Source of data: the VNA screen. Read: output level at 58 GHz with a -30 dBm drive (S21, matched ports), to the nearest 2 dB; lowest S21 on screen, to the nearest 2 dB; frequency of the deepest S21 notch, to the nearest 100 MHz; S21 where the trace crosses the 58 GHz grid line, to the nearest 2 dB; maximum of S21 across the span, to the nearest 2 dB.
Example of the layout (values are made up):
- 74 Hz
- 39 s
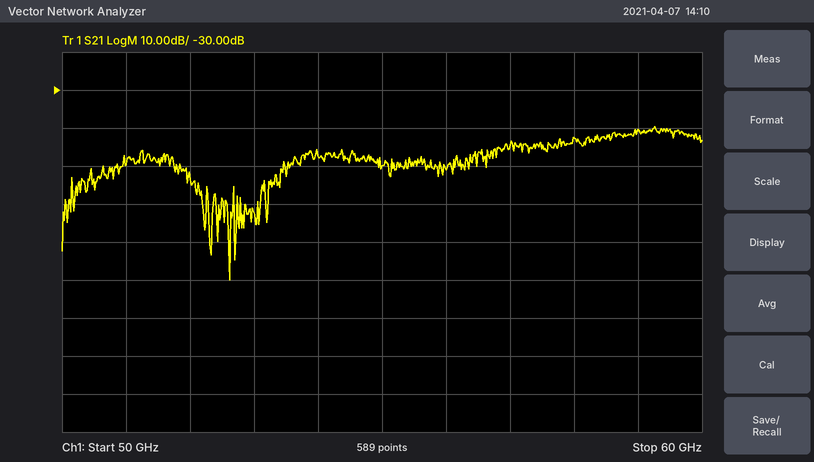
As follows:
- -72 dBm
- -80 dB
- 52.6 GHz
- -42 dB
- -40 dB
